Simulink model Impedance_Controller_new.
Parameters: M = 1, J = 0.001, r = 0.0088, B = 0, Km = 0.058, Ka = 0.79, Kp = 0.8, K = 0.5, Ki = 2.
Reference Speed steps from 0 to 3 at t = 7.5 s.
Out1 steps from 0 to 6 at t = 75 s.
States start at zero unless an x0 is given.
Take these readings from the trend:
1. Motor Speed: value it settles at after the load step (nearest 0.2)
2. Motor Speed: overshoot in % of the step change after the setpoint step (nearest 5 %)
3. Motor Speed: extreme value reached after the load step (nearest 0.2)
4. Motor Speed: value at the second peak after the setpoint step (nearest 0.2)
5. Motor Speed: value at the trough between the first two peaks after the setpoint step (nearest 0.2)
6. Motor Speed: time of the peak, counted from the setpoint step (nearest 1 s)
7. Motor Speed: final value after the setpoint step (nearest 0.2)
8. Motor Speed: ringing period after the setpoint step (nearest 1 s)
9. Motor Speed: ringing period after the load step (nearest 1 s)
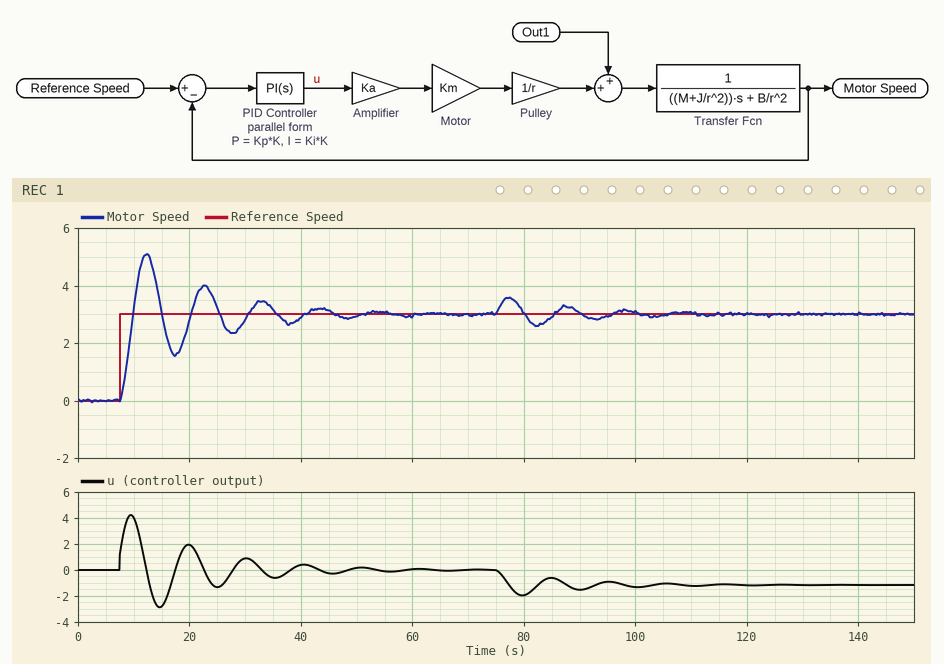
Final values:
3.0
70 %
3.6
4.0
1.6
5 s
3.0
10 s
10 s
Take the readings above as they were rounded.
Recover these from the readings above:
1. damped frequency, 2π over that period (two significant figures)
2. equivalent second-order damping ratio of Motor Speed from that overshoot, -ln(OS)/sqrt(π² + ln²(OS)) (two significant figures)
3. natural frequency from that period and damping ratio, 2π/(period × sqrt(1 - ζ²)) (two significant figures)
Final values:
0.63 rad/s
0.11
0.63 rad/s
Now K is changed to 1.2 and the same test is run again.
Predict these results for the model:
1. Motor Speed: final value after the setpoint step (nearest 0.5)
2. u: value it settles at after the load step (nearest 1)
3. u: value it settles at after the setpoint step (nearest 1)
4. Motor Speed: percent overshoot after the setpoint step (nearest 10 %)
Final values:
3.0
-1
0
60 %
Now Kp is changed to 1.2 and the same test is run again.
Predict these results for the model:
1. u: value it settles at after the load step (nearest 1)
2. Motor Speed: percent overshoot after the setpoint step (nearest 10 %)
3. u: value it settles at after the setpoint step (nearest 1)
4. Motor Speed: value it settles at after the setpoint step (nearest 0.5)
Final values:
-1
60 %
0
3.0
